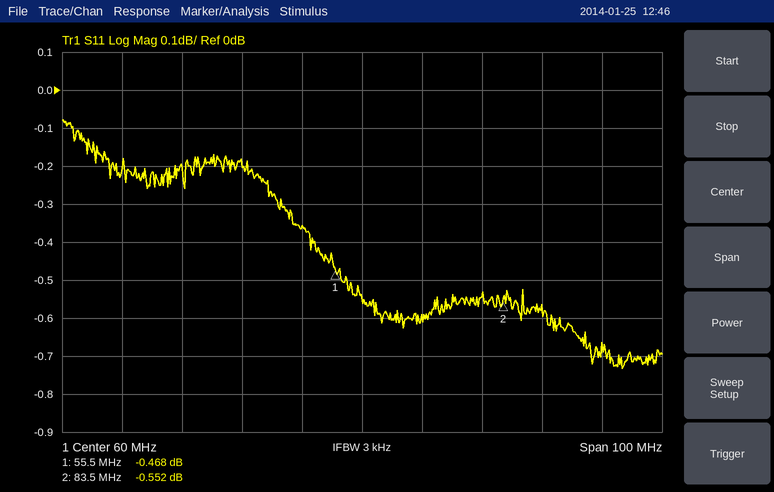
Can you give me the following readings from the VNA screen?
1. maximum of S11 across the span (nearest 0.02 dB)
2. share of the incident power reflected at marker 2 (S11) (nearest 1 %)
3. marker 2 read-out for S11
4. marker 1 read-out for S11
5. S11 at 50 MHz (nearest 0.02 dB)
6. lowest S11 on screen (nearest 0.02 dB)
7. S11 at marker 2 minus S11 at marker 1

-0.08 dB
88 %
-0.552 dB
-0.468 dB
-0.36 dB
-0.74 dB
-0.084 dB
